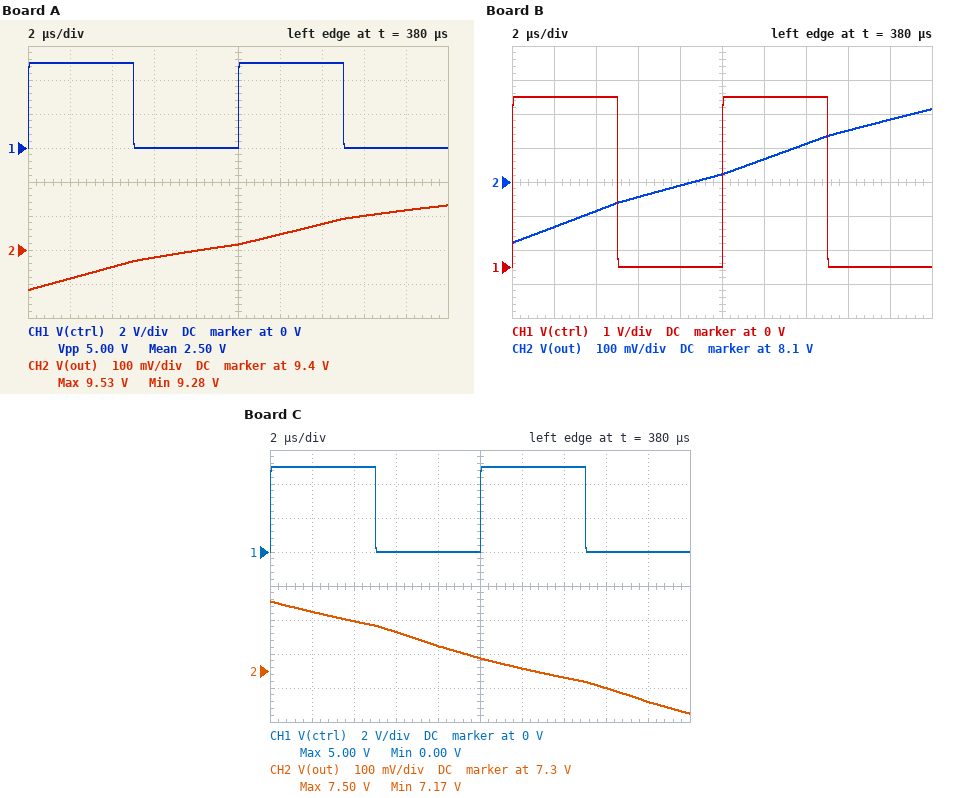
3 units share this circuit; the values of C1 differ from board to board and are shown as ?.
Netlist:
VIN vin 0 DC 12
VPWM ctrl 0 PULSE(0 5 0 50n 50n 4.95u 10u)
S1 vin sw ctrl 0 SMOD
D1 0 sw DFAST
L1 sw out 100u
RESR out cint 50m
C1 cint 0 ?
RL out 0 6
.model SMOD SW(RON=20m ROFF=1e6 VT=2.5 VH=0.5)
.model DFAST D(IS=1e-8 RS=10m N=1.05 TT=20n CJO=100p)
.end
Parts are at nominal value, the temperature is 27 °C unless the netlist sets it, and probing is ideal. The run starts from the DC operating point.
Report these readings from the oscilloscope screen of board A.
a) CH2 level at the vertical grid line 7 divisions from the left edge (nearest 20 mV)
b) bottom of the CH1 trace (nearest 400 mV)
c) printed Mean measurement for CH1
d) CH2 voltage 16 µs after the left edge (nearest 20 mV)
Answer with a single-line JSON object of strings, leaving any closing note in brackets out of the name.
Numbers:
{"CH2 level at the vertical grid line 7 divisions from the left edge": "9.48 V", "bottom of the CH1 trace": "0 V", "printed Mean measurement for CH1": "2.50 V", "CH2 voltage 16 µs after the left edge": "9.50 V"}
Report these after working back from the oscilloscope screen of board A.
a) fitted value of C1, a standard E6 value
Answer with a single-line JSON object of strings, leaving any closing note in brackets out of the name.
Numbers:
{"fitted value of C1, a standard E6 value": "220 µF"}
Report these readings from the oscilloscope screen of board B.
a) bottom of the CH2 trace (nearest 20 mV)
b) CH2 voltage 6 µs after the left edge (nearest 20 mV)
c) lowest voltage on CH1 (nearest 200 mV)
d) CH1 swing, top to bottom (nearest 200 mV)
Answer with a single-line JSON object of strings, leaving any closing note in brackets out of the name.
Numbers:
{"bottom of the CH2 trace": "7.92 V", "CH2 voltage 6 µs after the left edge": "8.06 V", "lowest voltage on CH1": "0 V", "CH1 swing, top to bottom": "5.0 V"}
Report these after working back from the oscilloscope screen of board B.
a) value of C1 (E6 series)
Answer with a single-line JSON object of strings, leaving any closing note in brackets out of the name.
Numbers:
{"value of C1": "330 µF"}
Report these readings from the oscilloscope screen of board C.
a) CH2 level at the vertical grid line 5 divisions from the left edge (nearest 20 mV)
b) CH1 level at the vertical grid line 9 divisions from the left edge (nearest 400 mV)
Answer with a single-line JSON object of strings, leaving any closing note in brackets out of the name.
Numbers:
{"CH2 level at the vertical grid line 5 divisions from the left edge": "7.34 V", "CH1 level at the vertical grid line 9 divisions from the left edge": "0 V"}
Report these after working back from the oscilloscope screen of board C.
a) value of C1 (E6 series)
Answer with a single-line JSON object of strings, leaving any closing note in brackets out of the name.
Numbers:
{"value of C1": "68 µF"}
